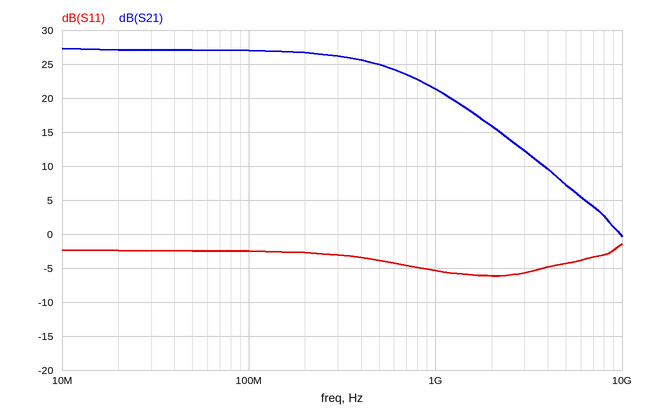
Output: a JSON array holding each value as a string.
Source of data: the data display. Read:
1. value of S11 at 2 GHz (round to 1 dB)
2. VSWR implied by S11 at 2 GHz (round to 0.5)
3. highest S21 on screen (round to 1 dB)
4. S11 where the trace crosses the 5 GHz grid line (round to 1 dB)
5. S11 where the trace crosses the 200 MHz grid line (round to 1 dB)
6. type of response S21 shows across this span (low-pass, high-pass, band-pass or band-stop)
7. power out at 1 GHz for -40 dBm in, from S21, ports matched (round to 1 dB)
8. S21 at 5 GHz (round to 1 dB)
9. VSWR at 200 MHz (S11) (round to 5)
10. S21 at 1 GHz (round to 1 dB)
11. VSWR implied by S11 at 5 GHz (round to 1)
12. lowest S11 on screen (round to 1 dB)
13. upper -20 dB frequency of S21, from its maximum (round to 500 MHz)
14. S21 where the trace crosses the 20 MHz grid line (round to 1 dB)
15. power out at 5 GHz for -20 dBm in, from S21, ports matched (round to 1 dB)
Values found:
["-6 dB", "3.0", "27 dB", "-4 dB", "-3 dB", "low-pass", "-19 dBm", "7 dB", "5", "21 dB", "4", "-6 dB", "5.0 GHz", "27 dB", "-13 dBm"]
